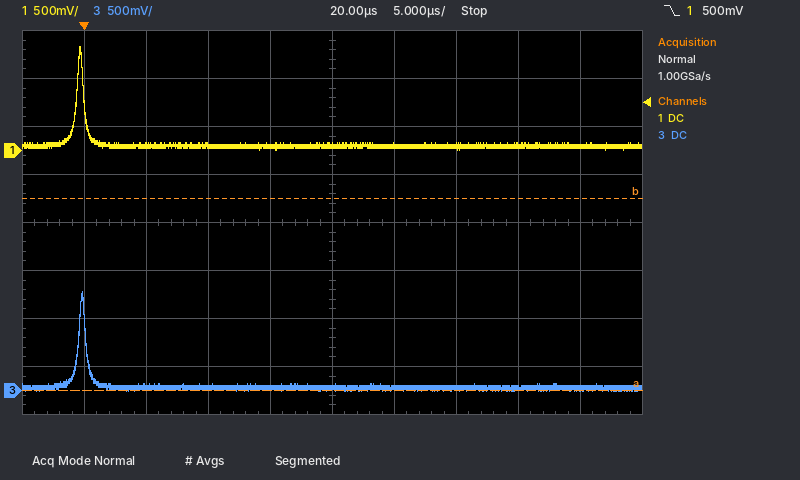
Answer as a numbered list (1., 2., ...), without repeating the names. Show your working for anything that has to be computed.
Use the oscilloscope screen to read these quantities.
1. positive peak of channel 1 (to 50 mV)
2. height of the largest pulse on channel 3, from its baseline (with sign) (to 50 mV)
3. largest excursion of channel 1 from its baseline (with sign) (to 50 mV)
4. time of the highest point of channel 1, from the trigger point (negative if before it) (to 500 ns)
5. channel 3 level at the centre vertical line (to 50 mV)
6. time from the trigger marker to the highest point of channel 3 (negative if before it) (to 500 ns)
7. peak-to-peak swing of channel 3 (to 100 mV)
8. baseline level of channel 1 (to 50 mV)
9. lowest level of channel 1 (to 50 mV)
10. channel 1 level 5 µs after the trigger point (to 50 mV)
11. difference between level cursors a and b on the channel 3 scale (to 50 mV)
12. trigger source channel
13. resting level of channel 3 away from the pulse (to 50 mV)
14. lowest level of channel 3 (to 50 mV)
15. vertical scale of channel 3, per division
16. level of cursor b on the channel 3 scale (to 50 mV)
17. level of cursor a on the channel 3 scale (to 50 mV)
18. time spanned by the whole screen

1. 1.10 V
2. +1.00 V
3. 1.10 V − (50 mV) = +1.05 V
4. -500 ns
5. 50 mV
6. 0.0 µs
7. 1.00 V
8. 50 mV
9. 0 mV
10. 50 mV
11. 2.00 V
12. channel 1
13. 50 mV
14. 0 mV
15. 500 mV
16. 2.00 V
17. 0 mV
18. 50 µs
